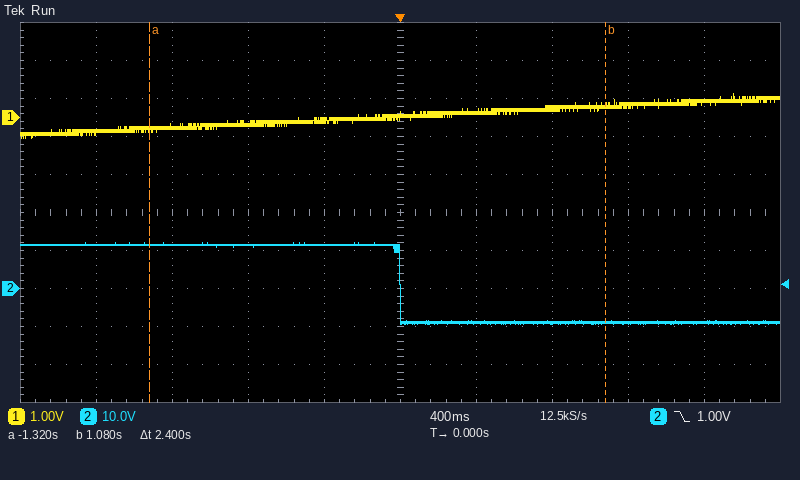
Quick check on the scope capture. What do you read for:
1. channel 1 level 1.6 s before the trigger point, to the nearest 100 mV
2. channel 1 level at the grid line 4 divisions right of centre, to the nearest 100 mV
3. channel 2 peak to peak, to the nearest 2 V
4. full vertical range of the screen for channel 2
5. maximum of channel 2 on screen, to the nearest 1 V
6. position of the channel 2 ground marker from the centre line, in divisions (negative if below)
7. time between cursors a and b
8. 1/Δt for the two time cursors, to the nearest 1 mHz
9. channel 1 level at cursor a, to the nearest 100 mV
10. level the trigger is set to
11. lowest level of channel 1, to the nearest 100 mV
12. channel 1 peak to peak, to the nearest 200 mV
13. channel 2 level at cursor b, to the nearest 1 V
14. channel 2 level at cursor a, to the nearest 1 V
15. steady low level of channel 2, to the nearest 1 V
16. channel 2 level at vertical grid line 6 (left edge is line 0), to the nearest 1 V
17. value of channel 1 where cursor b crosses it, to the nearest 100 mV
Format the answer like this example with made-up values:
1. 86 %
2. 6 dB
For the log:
1. -400 mV
2. 400 mV
3. 22 V
4. 100 V
5. 12 V
6. -2.0 div
7. 2.4 s
8. 417 mHz
9. -300 mV
10. 1.00 V
11. -600 mV
12. 1.2 V
13. -9 V
14. 11 V
15. -9 V
16. -9 V
17. 300 mV
